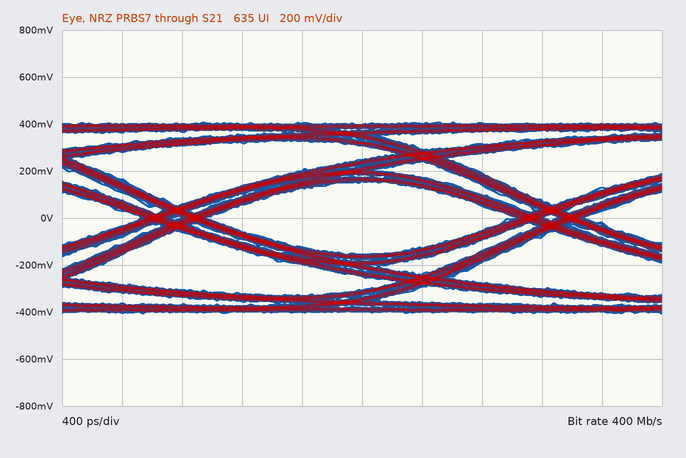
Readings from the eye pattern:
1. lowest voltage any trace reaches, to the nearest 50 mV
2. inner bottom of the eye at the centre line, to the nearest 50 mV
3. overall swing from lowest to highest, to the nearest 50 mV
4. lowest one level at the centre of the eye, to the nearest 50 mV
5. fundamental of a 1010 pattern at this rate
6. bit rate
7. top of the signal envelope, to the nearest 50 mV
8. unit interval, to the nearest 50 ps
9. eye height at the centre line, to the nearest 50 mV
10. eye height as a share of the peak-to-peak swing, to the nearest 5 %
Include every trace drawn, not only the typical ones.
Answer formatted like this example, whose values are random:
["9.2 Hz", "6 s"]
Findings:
["-400 mV", "-150 mV", "800 mV", "150 mV", "200 MHz", "400 Mb/s", "400 mV", "2.50 ns", "300 mV", "40 %"]
